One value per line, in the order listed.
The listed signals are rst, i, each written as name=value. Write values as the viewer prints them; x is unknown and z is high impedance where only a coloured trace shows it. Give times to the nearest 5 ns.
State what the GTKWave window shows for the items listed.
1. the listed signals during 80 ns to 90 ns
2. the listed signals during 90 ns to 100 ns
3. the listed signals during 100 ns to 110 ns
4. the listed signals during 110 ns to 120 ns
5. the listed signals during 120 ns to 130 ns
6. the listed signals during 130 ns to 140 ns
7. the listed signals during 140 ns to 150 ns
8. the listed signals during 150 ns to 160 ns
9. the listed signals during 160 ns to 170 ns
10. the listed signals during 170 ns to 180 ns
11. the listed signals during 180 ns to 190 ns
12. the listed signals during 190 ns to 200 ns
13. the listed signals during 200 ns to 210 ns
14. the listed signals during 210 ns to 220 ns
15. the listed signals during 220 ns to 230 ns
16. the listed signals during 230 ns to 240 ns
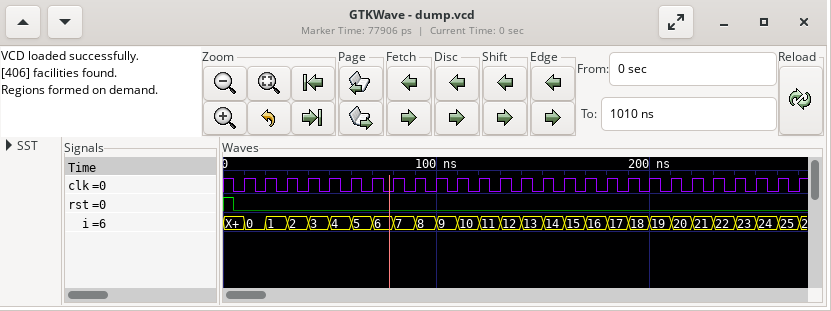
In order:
rst=0, i=7
rst=0, i=8
rst=0, i=9
rst=0, i=10
rst=0, i=11
rst=0, i=12
rst=0, i=13
rst=0, i=14
rst=0, i=15
rst=0, i=16
rst=0, i=17
rst=0, i=18
rst=0, i=19
rst=0, i=20
rst=0, i=21
rst=0, i=22
